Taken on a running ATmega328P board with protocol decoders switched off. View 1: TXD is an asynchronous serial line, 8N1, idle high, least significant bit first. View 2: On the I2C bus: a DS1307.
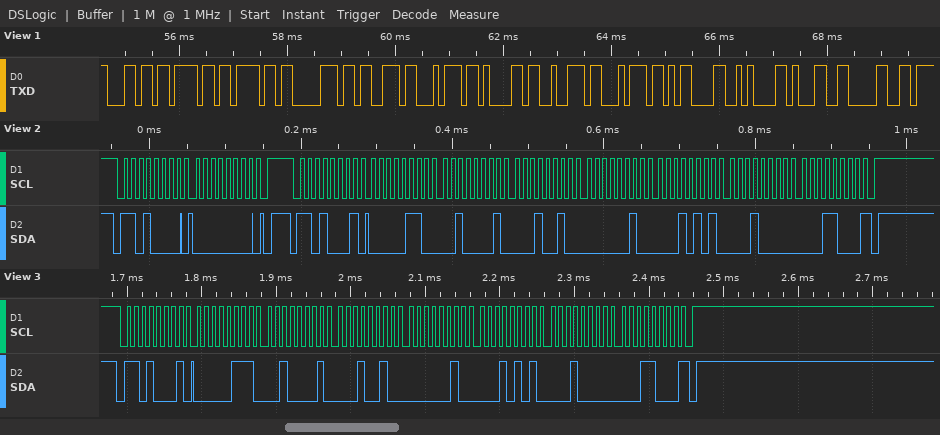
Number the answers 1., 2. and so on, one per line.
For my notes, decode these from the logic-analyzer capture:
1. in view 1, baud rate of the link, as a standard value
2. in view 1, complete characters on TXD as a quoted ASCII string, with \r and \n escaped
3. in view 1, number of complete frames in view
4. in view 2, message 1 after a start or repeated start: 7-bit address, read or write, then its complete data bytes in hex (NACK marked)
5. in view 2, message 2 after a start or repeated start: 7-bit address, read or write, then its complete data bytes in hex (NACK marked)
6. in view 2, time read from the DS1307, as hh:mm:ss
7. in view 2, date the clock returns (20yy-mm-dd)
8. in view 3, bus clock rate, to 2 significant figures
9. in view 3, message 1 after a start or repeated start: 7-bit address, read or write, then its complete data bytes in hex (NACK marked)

1. 9600 baud
2. "loopstart\r\n10"
3. 13
4. 0x68 write: 00
5. 0x68 read: 06 21 12 02 15 10 18 NACK
6. 12:21:06
7. 2018-10-15
8. 100 kHz
9. 0x68 read: 07 21 12 02 15 10 18 NACK
